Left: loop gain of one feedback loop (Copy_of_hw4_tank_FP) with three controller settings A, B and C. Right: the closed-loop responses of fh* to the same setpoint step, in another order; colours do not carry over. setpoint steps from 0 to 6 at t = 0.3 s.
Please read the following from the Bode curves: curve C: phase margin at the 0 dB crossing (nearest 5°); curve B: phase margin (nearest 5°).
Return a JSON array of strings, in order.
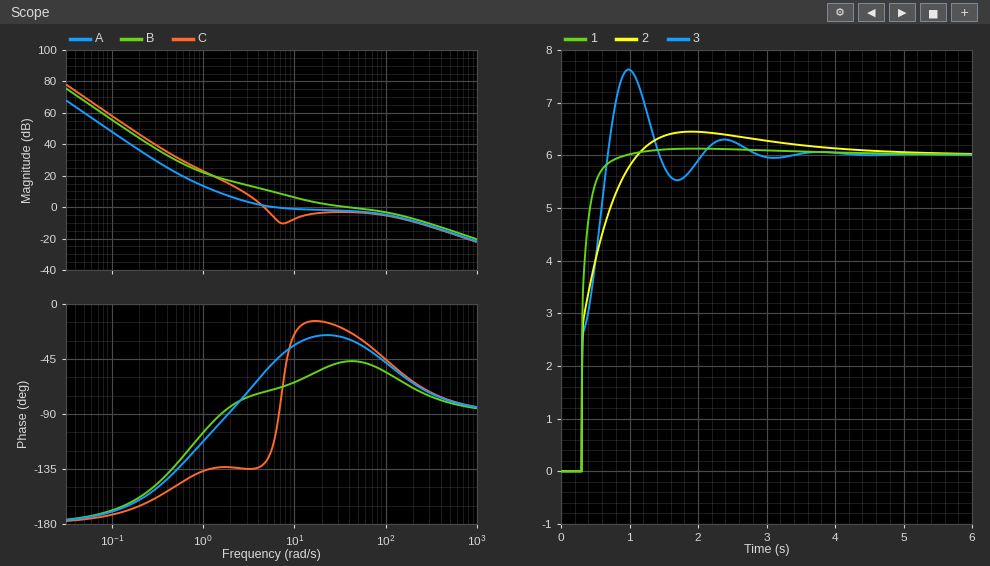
["50°", "135°"]
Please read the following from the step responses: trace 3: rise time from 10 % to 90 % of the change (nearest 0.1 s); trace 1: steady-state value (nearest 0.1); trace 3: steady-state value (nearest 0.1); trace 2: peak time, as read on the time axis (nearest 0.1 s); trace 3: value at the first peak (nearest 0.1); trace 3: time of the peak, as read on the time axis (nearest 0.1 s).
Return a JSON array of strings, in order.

["0.3 s", "6.0", "6.0", "1.9 s", "7.6", "1.0 s"]
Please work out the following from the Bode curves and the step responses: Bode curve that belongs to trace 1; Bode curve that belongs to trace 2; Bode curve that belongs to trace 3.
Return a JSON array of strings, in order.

["B", "A", "C"]
